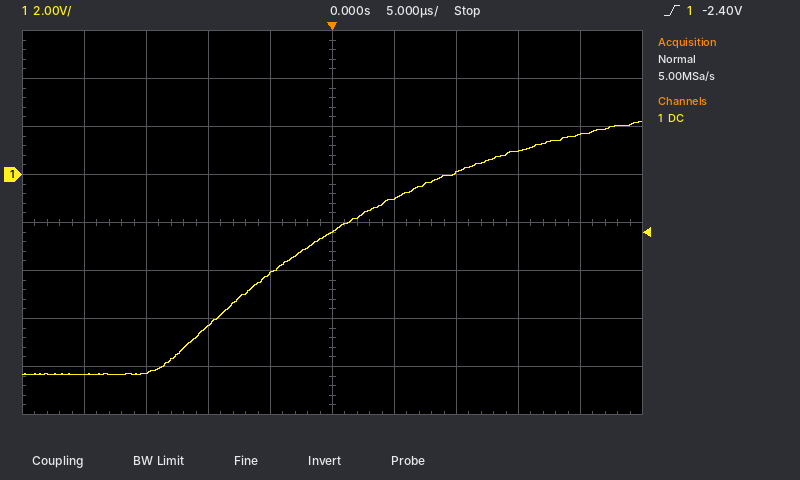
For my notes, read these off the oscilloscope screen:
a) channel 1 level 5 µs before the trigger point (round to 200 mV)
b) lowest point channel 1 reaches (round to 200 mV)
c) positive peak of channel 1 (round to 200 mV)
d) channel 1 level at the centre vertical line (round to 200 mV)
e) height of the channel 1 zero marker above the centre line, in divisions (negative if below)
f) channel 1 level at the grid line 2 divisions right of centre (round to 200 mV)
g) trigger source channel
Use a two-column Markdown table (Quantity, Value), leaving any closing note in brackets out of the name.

| Quantity | Value |
|---|---|
| channel 1 level 5 µs before the trigger point | -4.2 V |
| lowest point channel 1 reaches | -8.4 V |
| positive peak of channel 1 | 2.2 V |
| channel 1 level at the centre vertical line | -2.4 V |
| height of the channel 1 zero marker above the centre line, in divisions | +1.0 div |
| channel 1 level at the grid line 2 divisions right of centre | 0.0 V |
| trigger source channel | channel 1 |
